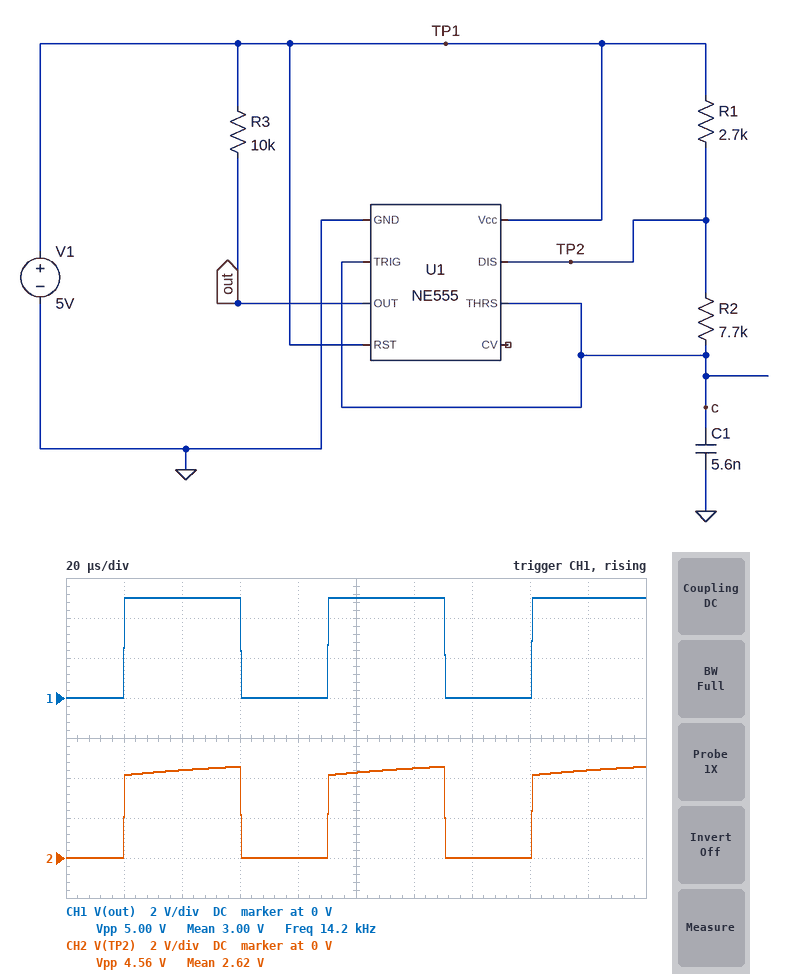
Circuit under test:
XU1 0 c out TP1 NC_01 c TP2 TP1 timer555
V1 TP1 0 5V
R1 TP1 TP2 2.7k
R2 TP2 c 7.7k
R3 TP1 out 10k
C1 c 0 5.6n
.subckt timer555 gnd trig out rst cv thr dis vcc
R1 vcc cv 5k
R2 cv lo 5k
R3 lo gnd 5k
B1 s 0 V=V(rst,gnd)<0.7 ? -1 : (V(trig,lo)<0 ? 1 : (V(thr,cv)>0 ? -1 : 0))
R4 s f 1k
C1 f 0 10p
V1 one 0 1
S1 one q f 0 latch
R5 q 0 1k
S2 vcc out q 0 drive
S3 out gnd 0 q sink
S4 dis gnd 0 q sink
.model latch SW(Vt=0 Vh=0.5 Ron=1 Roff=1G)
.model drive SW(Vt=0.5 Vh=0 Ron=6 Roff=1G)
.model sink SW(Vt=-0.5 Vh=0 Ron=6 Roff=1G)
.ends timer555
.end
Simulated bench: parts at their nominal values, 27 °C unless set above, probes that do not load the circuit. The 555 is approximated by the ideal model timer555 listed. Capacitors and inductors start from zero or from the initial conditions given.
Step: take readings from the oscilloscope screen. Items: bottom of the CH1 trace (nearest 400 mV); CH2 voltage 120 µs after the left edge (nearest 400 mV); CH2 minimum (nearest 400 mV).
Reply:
0 V
4.4 V
0 V
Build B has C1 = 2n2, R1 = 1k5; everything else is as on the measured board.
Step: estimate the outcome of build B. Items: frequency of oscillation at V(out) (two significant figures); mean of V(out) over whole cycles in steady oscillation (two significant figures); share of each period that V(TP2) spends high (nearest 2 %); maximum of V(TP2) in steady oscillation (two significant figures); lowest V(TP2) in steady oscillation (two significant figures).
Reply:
39 kHz
2.7 V
54 %
4.7 V
21 mV
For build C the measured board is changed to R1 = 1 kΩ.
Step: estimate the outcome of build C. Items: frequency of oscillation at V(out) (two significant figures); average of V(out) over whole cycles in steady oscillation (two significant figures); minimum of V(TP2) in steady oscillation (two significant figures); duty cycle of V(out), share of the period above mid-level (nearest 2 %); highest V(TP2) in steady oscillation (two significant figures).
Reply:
16 kHz
2.6 V
31 mV
52 %
4.8 V
